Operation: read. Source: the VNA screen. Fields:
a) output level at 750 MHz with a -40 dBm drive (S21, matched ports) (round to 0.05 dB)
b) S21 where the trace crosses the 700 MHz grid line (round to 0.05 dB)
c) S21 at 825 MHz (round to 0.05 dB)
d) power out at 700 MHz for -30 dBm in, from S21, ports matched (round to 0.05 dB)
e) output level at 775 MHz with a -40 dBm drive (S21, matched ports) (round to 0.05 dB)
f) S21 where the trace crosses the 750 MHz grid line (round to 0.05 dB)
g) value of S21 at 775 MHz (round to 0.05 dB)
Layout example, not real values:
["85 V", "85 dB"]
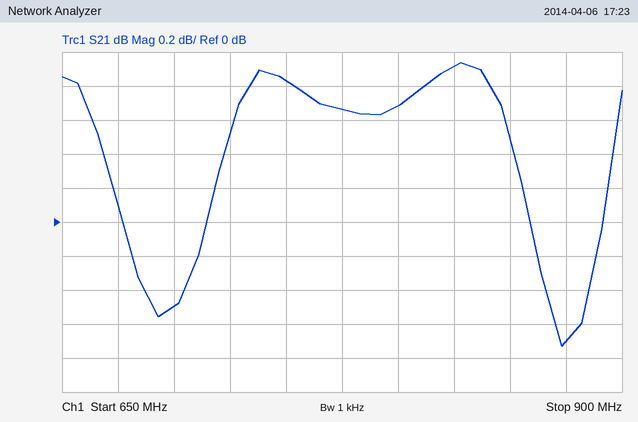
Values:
["-39.15 dBm", "-0.50 dB", "0.90 dB", "-30.50 dBm", "-39.35 dBm", "0.85 dB", "0.65 dB"]
